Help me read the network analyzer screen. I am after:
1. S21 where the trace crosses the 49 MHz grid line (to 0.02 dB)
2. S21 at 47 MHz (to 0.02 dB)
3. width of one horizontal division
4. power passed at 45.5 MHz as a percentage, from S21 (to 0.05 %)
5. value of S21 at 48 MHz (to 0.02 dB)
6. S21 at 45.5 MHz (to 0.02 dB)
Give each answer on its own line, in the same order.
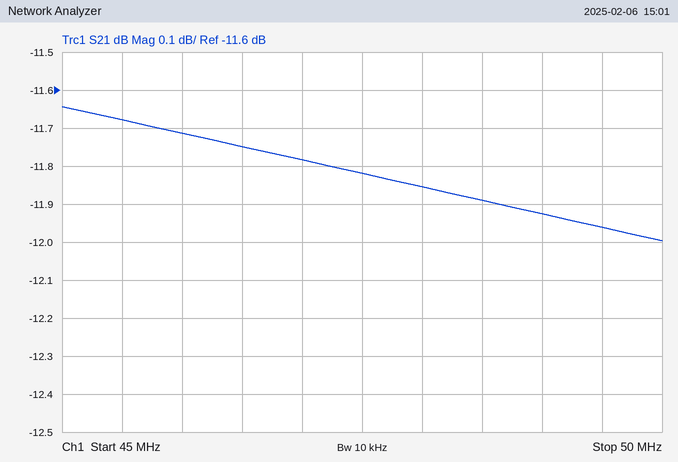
-11.92 dB
-11.78 dB
500 kHz
6.80 %
-11.86 dB
-11.68 dB
